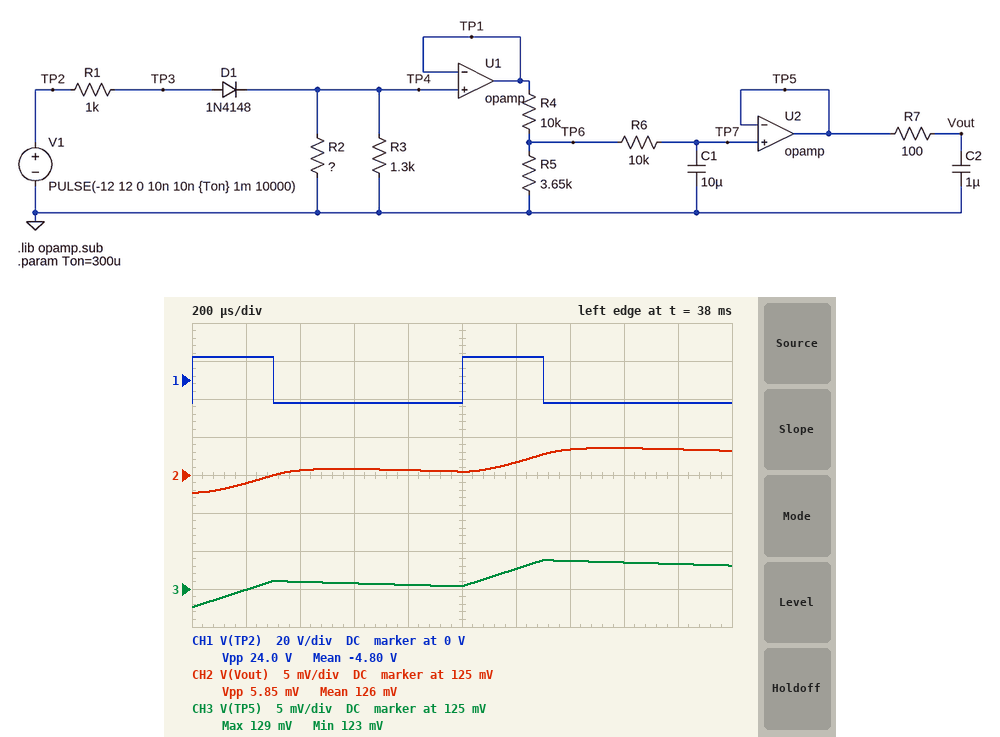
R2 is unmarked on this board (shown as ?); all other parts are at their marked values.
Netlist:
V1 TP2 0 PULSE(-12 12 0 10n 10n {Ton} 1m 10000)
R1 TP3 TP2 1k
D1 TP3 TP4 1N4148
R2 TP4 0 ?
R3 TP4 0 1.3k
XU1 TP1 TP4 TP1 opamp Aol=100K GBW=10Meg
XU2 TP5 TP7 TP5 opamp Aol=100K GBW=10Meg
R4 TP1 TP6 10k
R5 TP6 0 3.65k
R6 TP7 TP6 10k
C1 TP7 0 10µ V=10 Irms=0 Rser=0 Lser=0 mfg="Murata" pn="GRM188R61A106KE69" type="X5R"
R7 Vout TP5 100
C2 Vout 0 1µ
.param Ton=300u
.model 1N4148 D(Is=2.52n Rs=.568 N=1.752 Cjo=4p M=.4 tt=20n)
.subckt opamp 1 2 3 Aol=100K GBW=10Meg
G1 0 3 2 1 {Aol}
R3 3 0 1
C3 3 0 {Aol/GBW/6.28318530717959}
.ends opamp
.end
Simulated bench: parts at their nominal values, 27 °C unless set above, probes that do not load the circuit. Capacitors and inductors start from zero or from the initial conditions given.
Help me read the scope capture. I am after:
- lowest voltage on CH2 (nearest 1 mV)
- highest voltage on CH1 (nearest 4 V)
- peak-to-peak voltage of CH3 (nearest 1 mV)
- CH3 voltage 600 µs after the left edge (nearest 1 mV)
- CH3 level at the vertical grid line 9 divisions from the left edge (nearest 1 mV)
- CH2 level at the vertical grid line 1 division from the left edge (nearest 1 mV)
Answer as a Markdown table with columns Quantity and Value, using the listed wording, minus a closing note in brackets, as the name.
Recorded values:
| Quantity | Value |
|---|---|
| lowest voltage on CH2 | 123 mV |
| highest voltage on CH1 | 12 V |
| peak-to-peak voltage of CH3 | 6 mV |
| CH3 voltage 600 µs after the left edge | 126 mV |
| CH3 level at the vertical grid line 9 divisions from the left edge | 128 mV |
| CH2 level at the vertical grid line 1 division from the left edge | 124 mV |
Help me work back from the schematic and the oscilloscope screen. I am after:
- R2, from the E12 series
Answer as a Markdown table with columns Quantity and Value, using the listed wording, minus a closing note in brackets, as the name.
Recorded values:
| Quantity | Value |
|---|---|
| R2, from the E12 series | 6.8 kΩ |
